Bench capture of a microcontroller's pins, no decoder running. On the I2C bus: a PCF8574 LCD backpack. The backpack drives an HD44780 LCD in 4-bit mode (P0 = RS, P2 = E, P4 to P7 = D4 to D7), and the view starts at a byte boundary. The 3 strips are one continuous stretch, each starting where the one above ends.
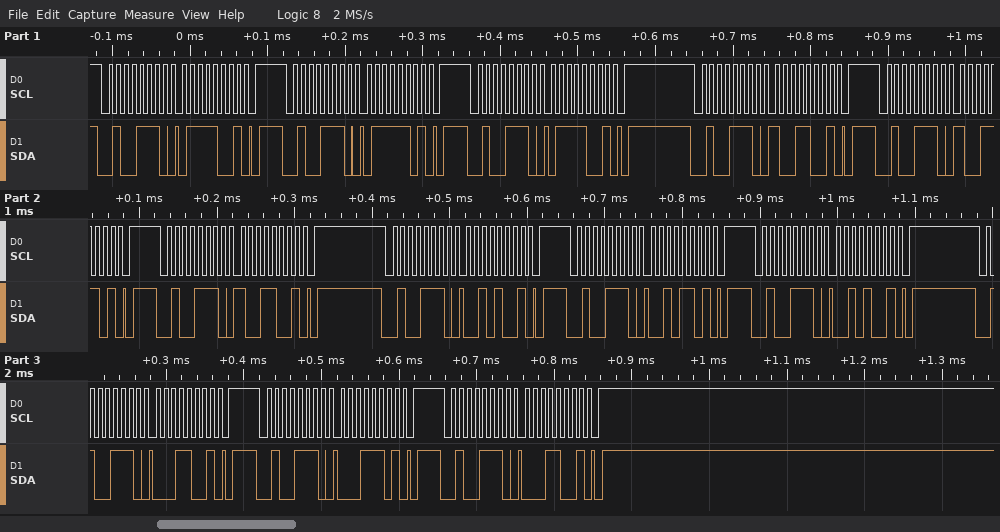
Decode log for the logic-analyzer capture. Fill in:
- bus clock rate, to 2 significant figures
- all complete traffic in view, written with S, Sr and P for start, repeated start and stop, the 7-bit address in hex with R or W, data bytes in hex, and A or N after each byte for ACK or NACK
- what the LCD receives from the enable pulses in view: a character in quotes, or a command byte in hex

100 kHz
S 27W A 79 A P S 27W A 7D A P S 27W A 79 A P S 27W A 99 A P S 27W A 9D A P S 27W A 99 A P S 27W A 29 A P S 27W A 2D A P S 27W A 29 A P S 27W A 19 A P S 27W A 1D A P S 27W A 19 A P
'y' '!'
